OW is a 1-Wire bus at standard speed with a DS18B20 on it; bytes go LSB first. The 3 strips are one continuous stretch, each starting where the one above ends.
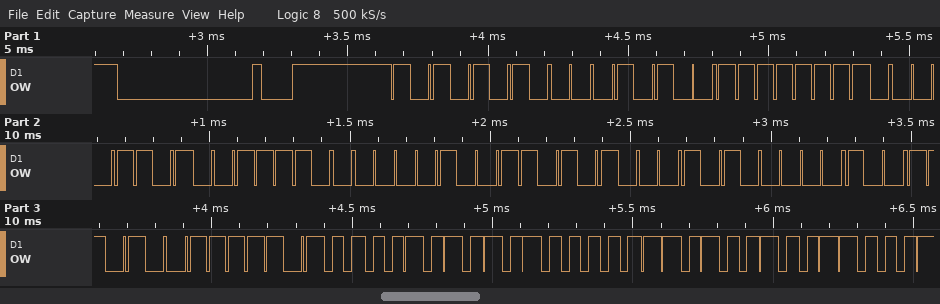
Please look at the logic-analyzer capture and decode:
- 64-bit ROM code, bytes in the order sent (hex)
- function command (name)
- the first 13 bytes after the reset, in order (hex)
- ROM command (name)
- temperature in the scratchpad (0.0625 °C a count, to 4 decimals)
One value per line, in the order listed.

28 FF B0 3C 90 15 05 59
Read Scratchpad
55 28 FF B0 3C 90 15 05 59 BE 50 05 4B
Match ROM
85.0000 °C
